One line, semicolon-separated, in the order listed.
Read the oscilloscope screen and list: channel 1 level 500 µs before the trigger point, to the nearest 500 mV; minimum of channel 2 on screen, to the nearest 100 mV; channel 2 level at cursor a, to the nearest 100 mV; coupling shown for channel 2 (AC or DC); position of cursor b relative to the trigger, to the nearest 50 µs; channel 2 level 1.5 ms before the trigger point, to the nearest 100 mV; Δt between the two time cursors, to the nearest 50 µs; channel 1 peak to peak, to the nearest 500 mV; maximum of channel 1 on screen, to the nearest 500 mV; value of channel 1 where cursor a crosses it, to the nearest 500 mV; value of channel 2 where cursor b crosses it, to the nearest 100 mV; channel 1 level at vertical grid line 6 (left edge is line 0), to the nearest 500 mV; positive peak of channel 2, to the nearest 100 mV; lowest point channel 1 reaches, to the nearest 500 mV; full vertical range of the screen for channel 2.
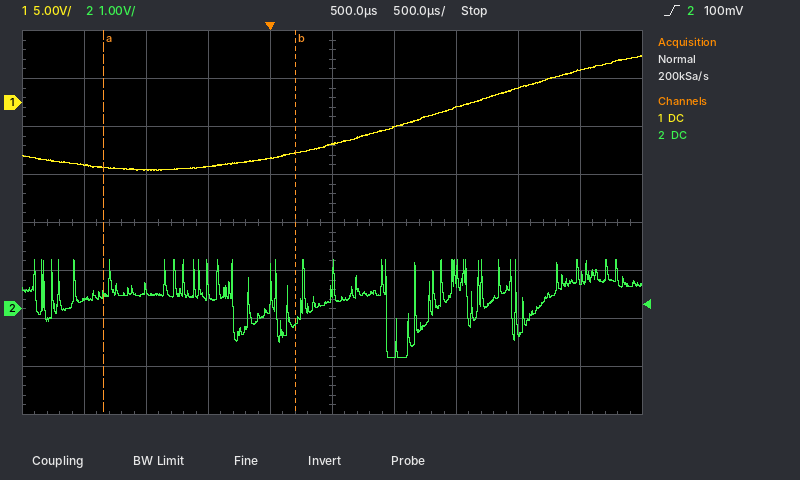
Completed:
-6.5 V; -1.0 V; 300 mV; DC; +200 µs; 200 mV; 1.55 ms; 12.0 V; 5.0 V; -6.5 V; -300 mV; -2.5 V; 1.0 V; -7.0 V; 8 V
